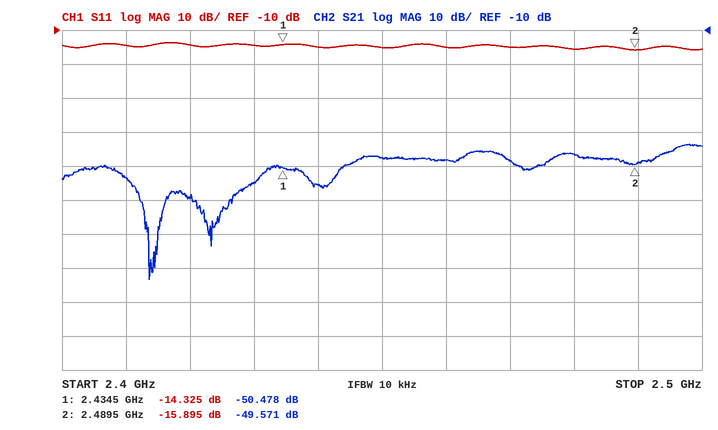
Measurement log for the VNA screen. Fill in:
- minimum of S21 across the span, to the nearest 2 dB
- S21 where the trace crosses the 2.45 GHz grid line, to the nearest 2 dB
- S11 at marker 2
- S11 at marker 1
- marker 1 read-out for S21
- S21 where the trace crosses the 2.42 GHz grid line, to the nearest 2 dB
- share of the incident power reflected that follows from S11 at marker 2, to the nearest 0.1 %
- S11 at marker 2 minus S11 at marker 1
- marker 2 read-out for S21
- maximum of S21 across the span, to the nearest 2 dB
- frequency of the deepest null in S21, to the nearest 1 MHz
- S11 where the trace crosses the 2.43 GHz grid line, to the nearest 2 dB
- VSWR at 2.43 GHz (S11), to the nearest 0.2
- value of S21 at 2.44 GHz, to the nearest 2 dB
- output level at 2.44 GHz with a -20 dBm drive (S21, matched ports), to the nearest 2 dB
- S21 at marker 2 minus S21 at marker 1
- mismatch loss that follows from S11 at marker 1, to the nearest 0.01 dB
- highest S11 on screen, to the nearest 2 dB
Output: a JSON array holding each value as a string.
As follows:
["-84 dB", "-48 dB", "-15.895 dB", "-14.325 dB", "-50.478 dB", "-60 dB", "2.6 %", "-1.570 dB", "-49.571 dB", "-44 dB", "2.414 GHz", "-14 dB", "1.4", "-56 dB", "-76 dBm", "0.907 dB", "0.16 dB", "-14 dB"]
